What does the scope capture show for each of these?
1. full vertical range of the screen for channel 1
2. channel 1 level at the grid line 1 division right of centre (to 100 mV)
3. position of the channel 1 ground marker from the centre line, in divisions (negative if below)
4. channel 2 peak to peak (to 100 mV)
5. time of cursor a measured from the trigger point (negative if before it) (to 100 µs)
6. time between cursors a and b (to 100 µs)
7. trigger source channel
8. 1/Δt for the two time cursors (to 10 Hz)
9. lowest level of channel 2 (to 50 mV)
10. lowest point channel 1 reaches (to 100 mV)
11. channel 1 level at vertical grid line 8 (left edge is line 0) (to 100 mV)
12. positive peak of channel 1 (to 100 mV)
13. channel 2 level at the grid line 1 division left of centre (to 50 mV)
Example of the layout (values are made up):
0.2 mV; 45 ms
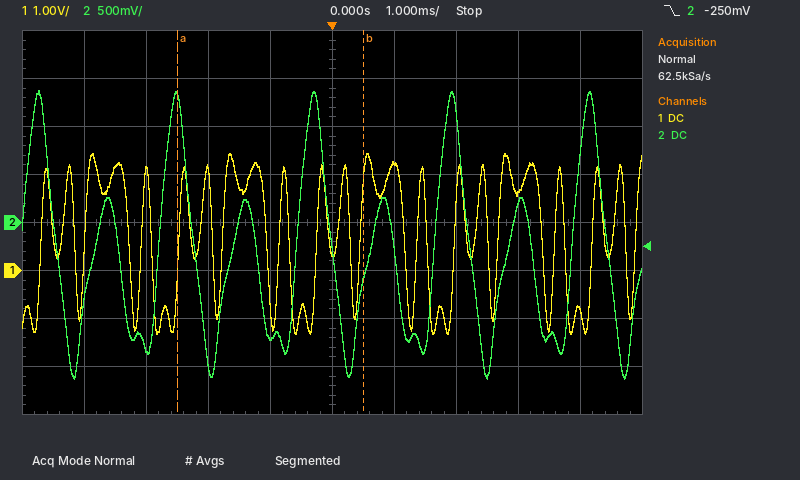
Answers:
8 V; 2.2 V; -1.0 div; 3.00 V; -2.5 ms; 3.0 ms; channel 2; 330 Hz; -1.60 V; -1.3 V; 1.6 V; 2.4 V; -1.20 V
